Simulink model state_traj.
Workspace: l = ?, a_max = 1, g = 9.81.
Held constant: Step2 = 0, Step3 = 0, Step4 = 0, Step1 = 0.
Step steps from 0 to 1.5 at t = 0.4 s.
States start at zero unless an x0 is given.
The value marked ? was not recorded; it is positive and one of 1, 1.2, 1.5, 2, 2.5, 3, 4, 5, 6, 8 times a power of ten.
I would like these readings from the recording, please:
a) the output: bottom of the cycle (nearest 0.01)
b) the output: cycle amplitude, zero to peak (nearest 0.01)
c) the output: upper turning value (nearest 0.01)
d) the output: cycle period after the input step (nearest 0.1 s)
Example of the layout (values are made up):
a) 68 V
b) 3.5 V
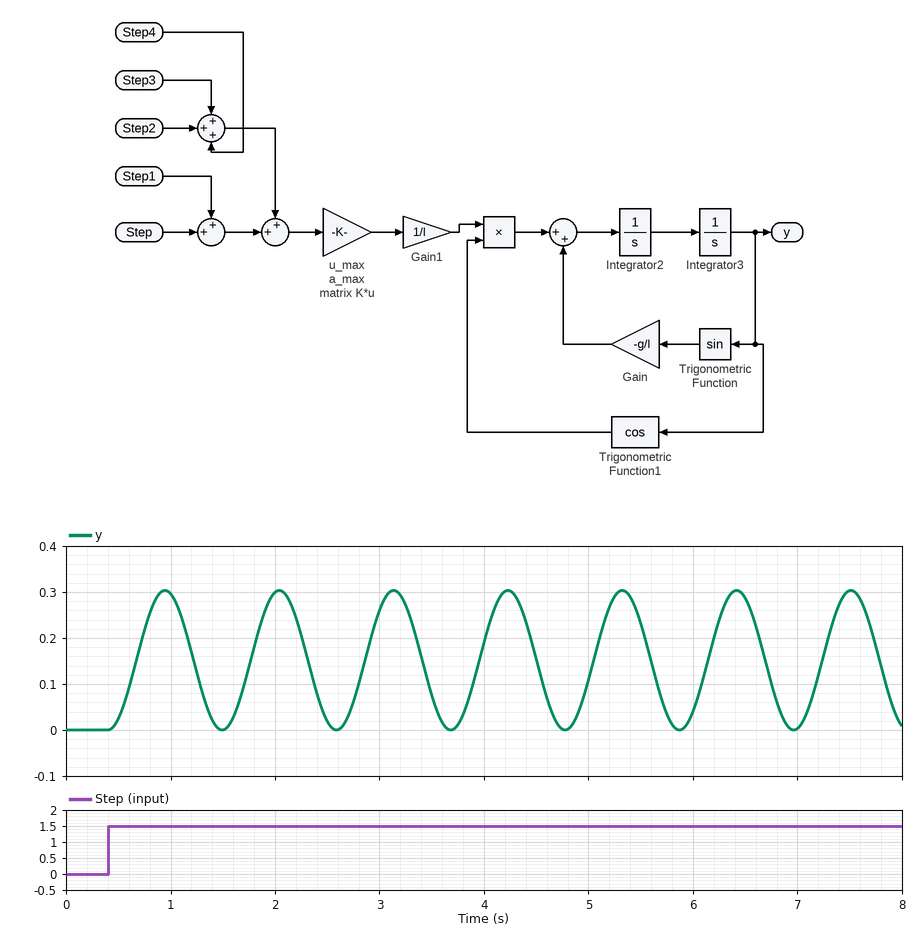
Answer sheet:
a) 0.00
b) 0.15
c) 0.30
d) 1.1 s
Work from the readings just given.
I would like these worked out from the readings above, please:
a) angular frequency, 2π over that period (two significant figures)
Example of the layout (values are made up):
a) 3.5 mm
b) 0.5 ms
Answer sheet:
a) 5.7 rad/s
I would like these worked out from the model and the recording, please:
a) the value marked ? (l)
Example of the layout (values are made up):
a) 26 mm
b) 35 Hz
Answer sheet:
a) 0.3
